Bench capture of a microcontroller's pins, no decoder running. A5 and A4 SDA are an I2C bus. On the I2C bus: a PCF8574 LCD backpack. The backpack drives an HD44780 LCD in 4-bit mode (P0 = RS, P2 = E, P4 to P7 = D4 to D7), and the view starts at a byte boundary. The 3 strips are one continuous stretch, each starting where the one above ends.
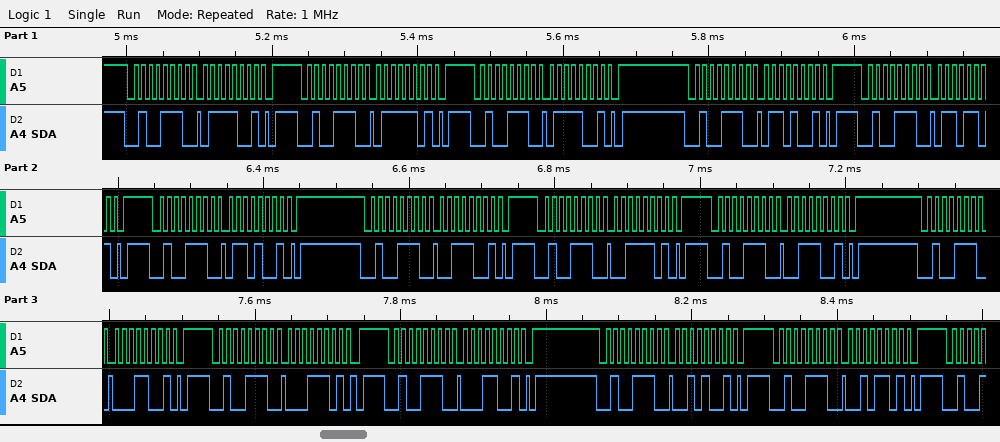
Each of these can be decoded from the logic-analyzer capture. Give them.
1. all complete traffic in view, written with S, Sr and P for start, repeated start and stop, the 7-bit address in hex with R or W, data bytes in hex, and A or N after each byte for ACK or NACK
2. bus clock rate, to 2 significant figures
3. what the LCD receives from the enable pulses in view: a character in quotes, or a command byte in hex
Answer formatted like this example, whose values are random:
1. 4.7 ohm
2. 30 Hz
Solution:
1. S 27W A 79 A P S 27W A 7D A P S 27W A 79 A P S 27W A 69 A P S 27W A 6D A P S 27W A 69 A P S 27W A 39 A P S 27W A 3D A P S 27W A 39 A P S 27W A 19 A P S 27W A 1D A P S 27W A 19 A P S 27W A 29 A P S 27W A 2D A P
2. 100 kHz
3. 'v' '1'
